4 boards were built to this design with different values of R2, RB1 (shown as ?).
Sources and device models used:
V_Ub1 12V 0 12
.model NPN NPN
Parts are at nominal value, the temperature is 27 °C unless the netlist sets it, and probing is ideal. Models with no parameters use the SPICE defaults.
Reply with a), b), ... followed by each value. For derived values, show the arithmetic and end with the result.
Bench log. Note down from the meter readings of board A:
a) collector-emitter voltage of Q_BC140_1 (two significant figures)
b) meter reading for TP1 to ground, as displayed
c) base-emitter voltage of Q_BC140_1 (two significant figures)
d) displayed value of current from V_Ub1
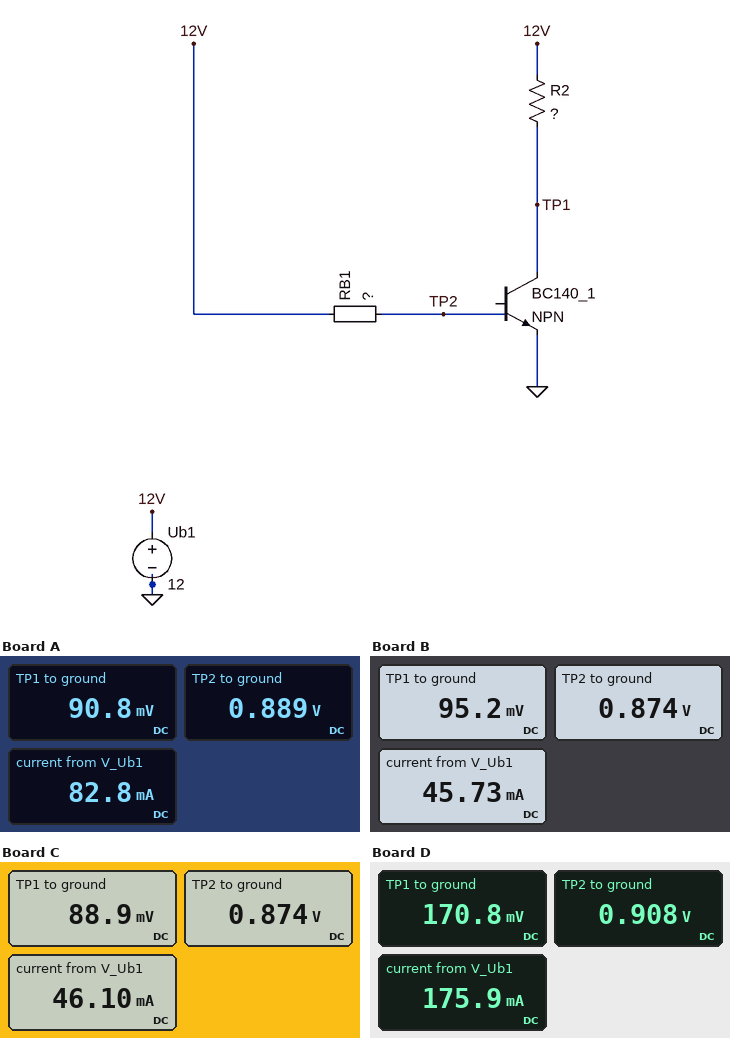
a) 90.8 mV = 91 mV
b) 90.8 mV
c) 889 mV = 890 mV
d) 82.8 mA
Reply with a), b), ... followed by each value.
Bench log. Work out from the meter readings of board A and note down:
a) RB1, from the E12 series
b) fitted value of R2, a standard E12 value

a) 3.3 kΩ
b) 150 Ω
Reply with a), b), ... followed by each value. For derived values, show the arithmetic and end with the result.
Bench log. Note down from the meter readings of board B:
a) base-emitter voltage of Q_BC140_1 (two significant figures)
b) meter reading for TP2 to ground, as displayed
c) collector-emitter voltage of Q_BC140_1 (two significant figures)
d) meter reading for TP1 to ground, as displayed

a) 874 mV = 870 mV
b) 0.874 V
c) 95.2 mV = 95 mV
d) 95.2 mV
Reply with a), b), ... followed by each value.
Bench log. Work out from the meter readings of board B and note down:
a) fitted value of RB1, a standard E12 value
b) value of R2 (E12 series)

a) 6.8 kΩ
b) 270 Ω
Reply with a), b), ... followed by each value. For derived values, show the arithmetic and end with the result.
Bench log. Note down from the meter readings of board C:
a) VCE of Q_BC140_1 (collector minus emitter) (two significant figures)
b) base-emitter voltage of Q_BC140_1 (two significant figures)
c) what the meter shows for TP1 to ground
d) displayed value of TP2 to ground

a) 88.9 mV = 89 mV
b) 874 mV = 870 mV
c) 88.9 mV
d) 0.874 V
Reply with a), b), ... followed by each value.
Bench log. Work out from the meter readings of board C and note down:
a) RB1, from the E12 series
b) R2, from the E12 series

a) 5.6 kΩ
b) 270 Ω
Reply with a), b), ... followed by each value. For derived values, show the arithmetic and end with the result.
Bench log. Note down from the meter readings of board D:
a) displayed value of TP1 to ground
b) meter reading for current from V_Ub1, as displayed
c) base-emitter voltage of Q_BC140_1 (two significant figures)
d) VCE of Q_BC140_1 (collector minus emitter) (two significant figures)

a) 170.8 mV
b) 175.9 mA
c) 908 mV = 910 mV
d) 170.8 mV = 170 mV
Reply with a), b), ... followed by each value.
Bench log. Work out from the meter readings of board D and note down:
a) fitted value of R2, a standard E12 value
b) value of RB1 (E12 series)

a) 68 Ω
b) 5.6 kΩ
